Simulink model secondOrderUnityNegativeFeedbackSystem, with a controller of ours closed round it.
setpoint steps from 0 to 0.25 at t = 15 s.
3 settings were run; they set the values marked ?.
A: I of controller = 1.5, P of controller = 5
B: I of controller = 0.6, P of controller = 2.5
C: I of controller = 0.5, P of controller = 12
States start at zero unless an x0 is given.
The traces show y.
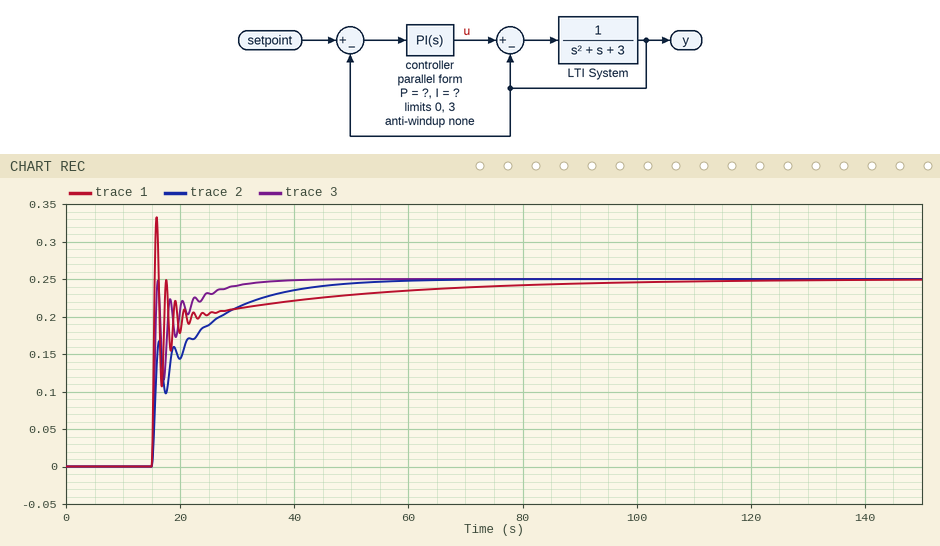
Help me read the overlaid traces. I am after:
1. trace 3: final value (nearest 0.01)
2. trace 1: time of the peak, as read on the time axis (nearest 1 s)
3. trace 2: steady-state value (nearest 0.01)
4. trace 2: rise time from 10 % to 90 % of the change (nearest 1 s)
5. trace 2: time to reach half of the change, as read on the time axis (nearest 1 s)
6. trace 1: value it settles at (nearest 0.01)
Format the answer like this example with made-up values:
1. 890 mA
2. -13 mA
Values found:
1. 0.25
2. 16 s
3. 0.25
4. 19 s
5. 16 s
6. 0.25
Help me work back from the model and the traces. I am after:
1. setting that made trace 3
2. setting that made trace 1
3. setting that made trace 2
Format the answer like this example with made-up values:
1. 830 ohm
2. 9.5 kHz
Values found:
1. A
2. C
3. B
